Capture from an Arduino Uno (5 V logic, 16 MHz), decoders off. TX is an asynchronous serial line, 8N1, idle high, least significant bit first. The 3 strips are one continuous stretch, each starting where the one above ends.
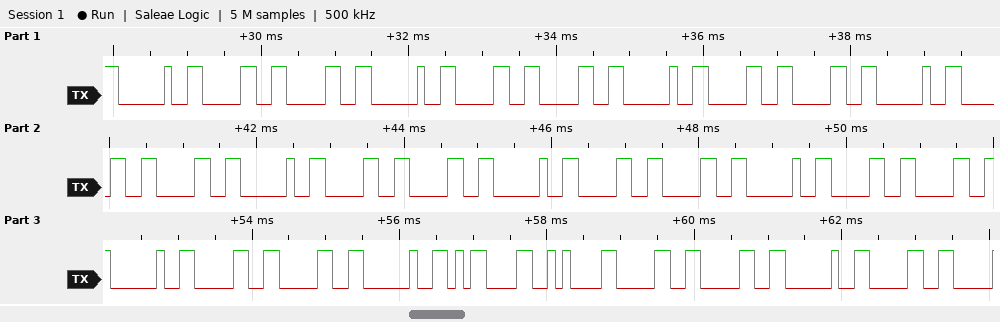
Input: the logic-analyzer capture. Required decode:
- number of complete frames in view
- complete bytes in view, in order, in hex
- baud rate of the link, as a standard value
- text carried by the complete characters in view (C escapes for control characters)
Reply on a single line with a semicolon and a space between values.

31; 20 30 30 20 30 30 20 30 30 20 30 30 20 30 30 20 30 30 20 30 30 20 30 30 20 0D 0A 30 30 20 30; 9600 baud; " 00 00 00 00 00 00 00 00 \r\n00 0"
